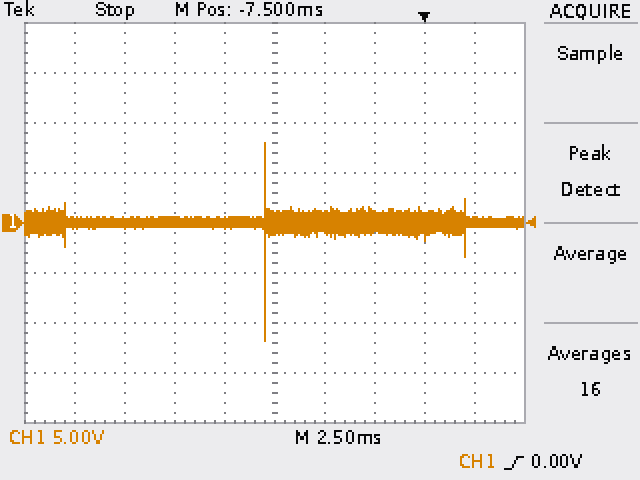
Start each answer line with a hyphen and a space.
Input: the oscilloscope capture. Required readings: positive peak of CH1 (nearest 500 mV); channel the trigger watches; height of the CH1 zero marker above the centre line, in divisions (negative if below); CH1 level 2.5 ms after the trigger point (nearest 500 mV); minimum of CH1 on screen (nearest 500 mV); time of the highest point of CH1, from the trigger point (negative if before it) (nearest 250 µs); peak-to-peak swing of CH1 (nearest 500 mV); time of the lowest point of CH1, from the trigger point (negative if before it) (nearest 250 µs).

- 8.0 V
- CH1
- 0.0 div
- 0.0 V
- -12.0 V
- -8.00 ms
- 20.0 V
- -8.00 ms
